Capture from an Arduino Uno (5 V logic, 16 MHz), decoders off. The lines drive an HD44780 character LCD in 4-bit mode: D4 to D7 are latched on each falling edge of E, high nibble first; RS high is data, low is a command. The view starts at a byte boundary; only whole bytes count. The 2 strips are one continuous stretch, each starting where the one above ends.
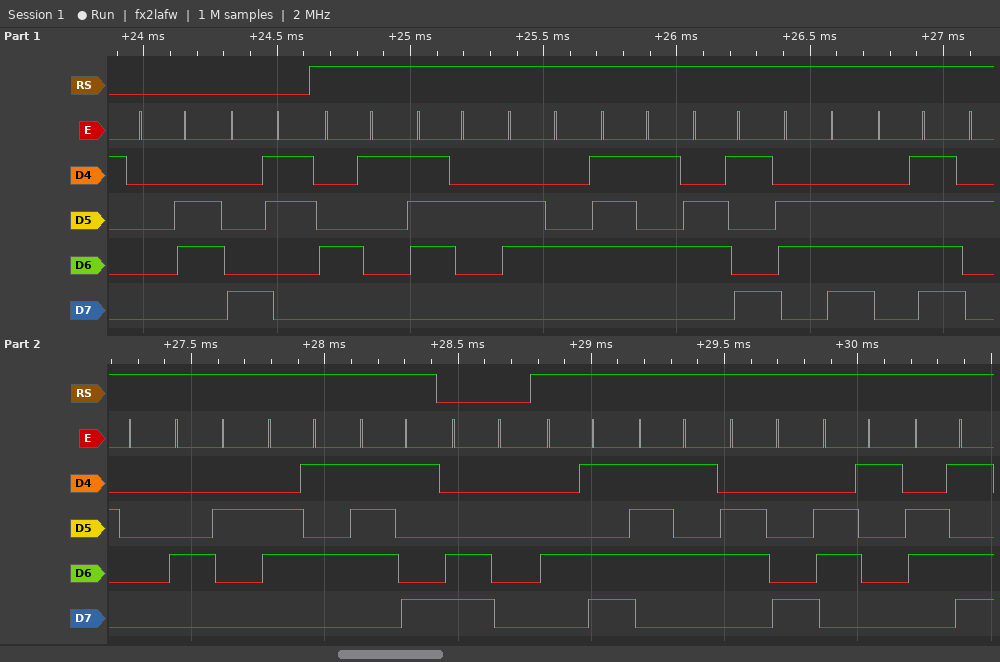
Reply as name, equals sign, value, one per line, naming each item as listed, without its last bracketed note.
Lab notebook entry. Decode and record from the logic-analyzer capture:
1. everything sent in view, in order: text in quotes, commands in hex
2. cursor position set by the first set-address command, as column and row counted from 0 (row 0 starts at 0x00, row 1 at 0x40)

everything sent in view, in order: text in quotes, commands in hex = 0x06 0x83 "Arduino Bey" 0xC0 "Muham"
cursor position set by the first set-address command, as column and row counted from 0 = column 3, row 0
